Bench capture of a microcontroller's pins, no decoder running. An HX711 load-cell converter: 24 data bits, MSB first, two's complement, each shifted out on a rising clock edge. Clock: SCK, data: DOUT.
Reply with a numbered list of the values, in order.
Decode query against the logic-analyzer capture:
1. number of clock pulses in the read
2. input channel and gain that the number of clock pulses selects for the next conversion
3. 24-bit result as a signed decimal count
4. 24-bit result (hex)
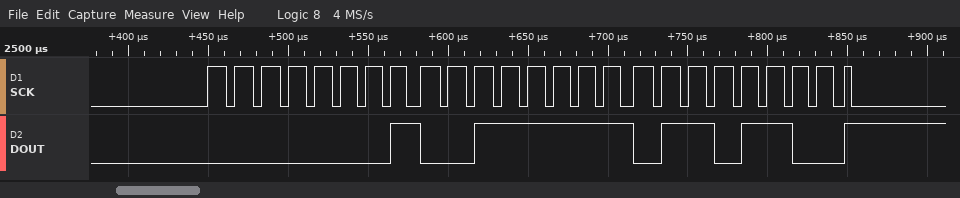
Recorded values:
1. 25
2. channel A, gain 128
3. 81772
4. 0x013F6C
